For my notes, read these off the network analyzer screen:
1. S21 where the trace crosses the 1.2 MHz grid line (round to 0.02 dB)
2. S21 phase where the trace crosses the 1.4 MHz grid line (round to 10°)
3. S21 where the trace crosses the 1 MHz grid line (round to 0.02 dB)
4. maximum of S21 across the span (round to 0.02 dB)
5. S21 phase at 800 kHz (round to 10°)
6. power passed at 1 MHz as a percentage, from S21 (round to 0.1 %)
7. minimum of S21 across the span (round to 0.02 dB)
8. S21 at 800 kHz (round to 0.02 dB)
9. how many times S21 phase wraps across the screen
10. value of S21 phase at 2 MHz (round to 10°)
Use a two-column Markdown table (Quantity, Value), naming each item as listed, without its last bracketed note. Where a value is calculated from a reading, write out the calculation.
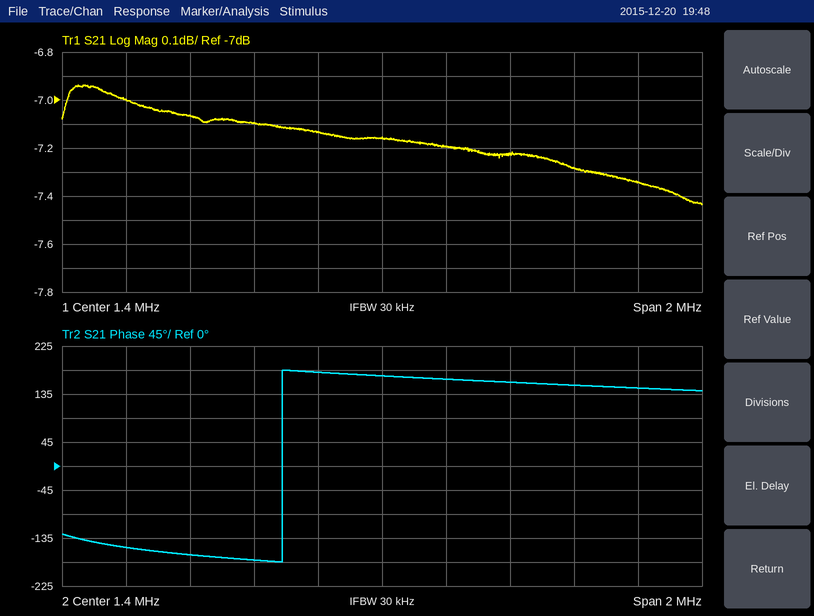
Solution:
| Quantity | Value |
|---|---|
| S21 where the trace crosses the 1.2 MHz grid line | -7.14 dB |
| S21 phase where the trace crosses the 1.4 MHz grid line | 170° |
| S21 where the trace crosses the 1 MHz grid line | -7.10 dB |
| maximum of S21 across the span | -6.94 dB |
| S21 phase at 800 kHz | -170° |
| power passed at 1 MHz as a percentage, from S21 | 10^(-7.1/10) ≈ 19.5 % |
| minimum of S21 across the span | -7.44 dB |
| S21 at 800 kHz | -7.06 dB |
| how many times S21 phase wraps across the screen | 1 |
| value of S21 phase at 2 MHz | 150° |
